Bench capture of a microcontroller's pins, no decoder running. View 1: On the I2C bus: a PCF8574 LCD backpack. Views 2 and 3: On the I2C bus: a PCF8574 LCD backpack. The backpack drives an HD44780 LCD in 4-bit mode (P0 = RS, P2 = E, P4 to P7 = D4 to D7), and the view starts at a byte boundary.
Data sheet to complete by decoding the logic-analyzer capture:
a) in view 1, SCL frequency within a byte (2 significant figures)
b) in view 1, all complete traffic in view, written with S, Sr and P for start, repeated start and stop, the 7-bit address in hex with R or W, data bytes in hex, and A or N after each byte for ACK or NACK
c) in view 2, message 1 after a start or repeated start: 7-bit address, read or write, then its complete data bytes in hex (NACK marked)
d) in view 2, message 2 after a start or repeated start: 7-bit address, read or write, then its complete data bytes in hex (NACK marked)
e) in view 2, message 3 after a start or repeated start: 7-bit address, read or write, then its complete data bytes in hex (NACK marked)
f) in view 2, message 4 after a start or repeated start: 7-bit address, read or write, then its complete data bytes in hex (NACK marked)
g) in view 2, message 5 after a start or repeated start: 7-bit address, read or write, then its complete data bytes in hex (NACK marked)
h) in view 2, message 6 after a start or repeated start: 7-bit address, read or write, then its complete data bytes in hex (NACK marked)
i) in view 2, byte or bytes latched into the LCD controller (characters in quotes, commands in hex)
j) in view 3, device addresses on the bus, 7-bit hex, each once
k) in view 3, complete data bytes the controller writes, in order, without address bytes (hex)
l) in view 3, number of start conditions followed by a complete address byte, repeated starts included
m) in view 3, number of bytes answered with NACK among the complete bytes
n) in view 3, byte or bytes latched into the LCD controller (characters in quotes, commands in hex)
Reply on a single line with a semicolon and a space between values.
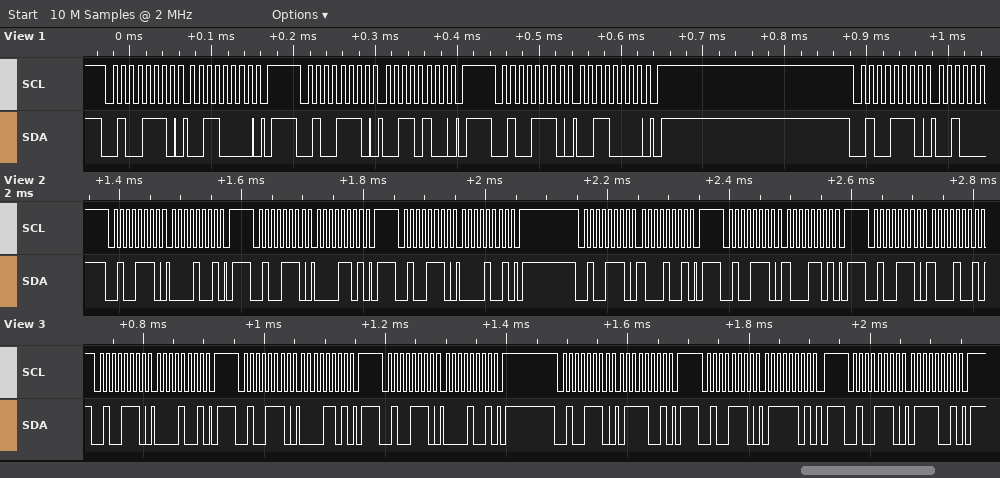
100 kHz; S 27W A 30 A P S 27W A 34 A P S 27W A 30 A P S 27W A; 0x27 write: 09; 0x27 write: 0D; 0x27 write: 09; 0x27 write: 89; 0x27 write: 8D; 0x27 write: 89; data 0x08; 0x27; 09 0D 09 79 7D 79; 6; 0; data 0x07
